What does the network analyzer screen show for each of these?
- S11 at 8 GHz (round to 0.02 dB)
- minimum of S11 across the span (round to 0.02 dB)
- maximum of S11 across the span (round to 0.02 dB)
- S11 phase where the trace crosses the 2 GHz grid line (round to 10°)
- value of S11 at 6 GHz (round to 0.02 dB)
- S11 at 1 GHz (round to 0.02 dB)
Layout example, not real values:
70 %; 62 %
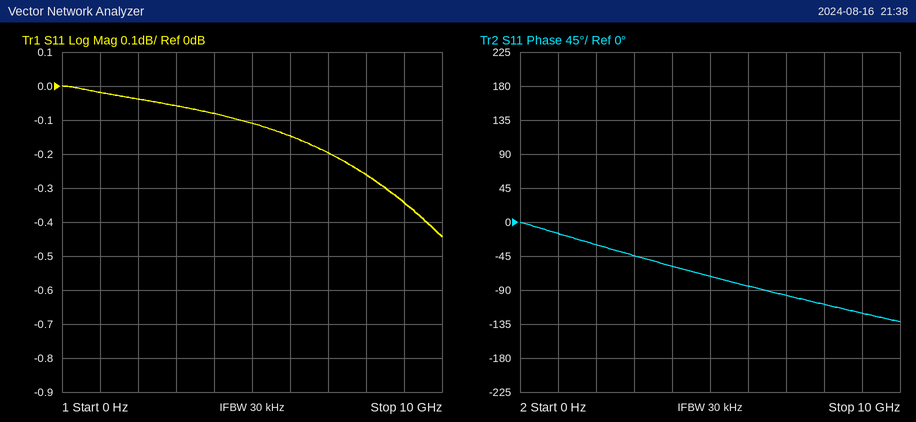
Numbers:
-0.26 dB; -0.44 dB; 0.00 dB; -30°; -0.14 dB; -0.02 dB
